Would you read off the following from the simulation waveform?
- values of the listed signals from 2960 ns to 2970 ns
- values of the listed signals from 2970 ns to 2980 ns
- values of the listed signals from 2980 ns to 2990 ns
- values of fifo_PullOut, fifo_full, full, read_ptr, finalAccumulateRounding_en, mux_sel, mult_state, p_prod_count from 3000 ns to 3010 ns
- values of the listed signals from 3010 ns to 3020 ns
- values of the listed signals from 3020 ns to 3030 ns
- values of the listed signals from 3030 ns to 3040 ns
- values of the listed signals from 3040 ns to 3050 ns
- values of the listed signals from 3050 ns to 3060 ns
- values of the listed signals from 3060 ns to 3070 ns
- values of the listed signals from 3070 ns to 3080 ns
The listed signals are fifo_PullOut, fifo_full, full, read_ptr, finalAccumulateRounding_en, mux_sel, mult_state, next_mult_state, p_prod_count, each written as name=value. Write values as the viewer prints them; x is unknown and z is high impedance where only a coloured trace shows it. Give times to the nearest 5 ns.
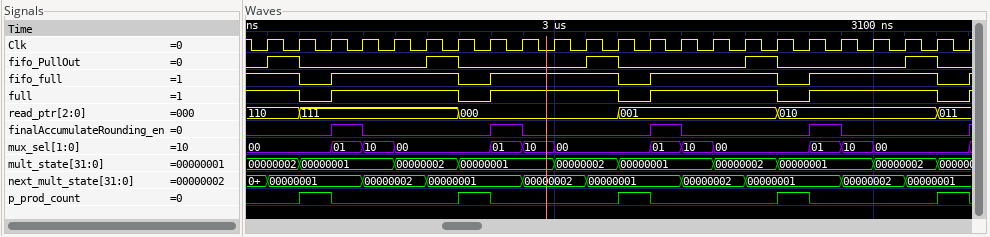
fifo_PullOut=1, fifo_full=1, full=1, read_ptr=111, finalAccumulateRounding_en=0, mux_sel=00, mult_state=00000002, next_mult_state=00000001, p_prod_count=0
fifo_PullOut=0, fifo_full=0, full=0, read_ptr=000, finalAccumulateRounding_en=0, mux_sel=00, mult_state=00000001, next_mult_state=00000001, p_prod_count=1
fifo_PullOut=0, fifo_full=1, full=1, read_ptr=000, finalAccumulateRounding_en=1, mux_sel=01, mult_state=00000001, next_mult_state=00000001, p_prod_count=0
fifo_PullOut=0, fifo_full=1, full=1, read_ptr=000, finalAccumulateRounding_en=0, mux_sel=00, mult_state=00000002, p_prod_count=0
fifo_PullOut=1, fifo_full=1, full=1, read_ptr=000, finalAccumulateRounding_en=0, mux_sel=00, mult_state=00000002, next_mult_state=00000001, p_prod_count=0
fifo_PullOut=0, fifo_full=0, full=0, read_ptr=001, finalAccumulateRounding_en=0, mux_sel=00, mult_state=00000001, next_mult_state=00000001, p_prod_count=1
fifo_PullOut=0, fifo_full=1, full=1, read_ptr=001, finalAccumulateRounding_en=1, mux_sel=01, mult_state=00000001, next_mult_state=00000001, p_prod_count=0
fifo_PullOut=0, fifo_full=1, full=1, read_ptr=001, finalAccumulateRounding_en=0, mux_sel=10, mult_state=00000001, next_mult_state=00000002, p_prod_count=0
fifo_PullOut=0, fifo_full=1, full=1, read_ptr=001, finalAccumulateRounding_en=0, mux_sel=00, mult_state=00000002, next_mult_state=00000002, p_prod_count=0
fifo_PullOut=1, fifo_full=1, full=1, read_ptr=001, finalAccumulateRounding_en=0, mux_sel=00, mult_state=00000002, next_mult_state=00000001, p_prod_count=0
fifo_PullOut=0, fifo_full=0, full=0, read_ptr=010, finalAccumulateRounding_en=0, mux_sel=00, mult_state=00000001, next_mult_state=00000001, p_prod_count=1
